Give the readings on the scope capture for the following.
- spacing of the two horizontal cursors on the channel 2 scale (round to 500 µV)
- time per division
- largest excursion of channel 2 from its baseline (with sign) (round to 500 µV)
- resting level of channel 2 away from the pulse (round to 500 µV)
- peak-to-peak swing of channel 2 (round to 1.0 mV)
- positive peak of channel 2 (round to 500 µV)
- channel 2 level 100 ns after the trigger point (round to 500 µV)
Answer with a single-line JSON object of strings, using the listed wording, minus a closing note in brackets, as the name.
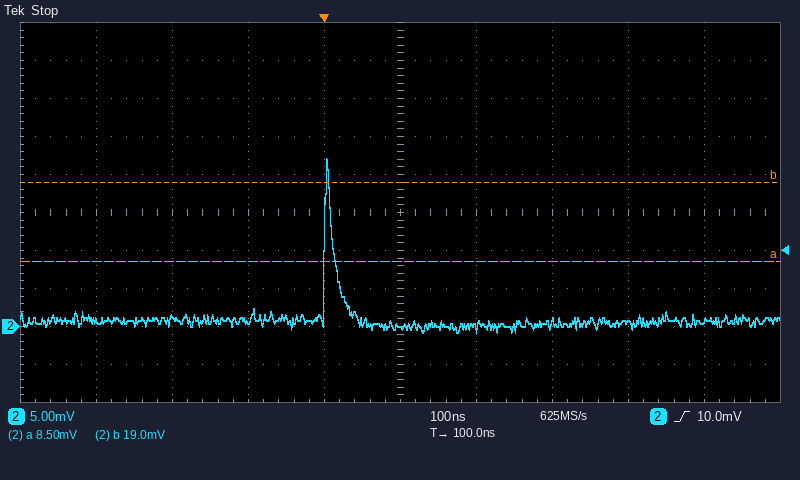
{"spacing of the two horizontal cursors on the channel 2 scale": "10.5 mV", "time per division": "100 ns", "largest excursion of channel 2 from its baseline (with sign)": "+21.5 mV", "resting level of channel 2 away from the pulse": "500 µV", "peak-to-peak swing of channel 2": "23.0 mV", "positive peak of channel 2": "22.0 mV", "channel 2 level 100 ns after the trigger point": "0.0 mV"}
